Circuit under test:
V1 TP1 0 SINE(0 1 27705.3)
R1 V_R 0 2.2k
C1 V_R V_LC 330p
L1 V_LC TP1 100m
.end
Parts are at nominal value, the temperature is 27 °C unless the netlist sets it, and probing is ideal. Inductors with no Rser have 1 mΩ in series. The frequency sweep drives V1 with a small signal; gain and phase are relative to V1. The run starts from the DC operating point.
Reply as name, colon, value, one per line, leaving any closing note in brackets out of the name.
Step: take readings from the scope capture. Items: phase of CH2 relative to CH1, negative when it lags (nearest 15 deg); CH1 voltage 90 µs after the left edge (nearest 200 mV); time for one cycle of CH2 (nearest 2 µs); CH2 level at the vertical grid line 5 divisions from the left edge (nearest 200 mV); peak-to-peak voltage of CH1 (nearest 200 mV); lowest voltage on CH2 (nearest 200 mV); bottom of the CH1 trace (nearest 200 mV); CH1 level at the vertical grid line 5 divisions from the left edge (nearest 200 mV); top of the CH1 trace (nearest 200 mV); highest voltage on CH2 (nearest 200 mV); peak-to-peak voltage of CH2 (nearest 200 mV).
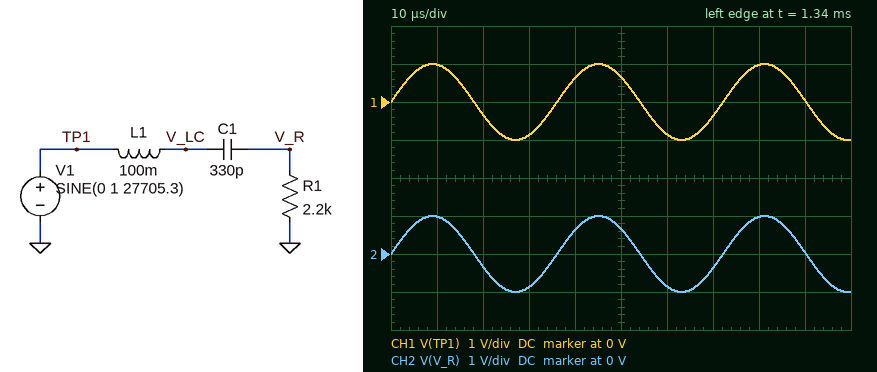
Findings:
phase of CH2 relative to CH1, negative when it lags: 0 deg
CH1 voltage 90 µs after the left edge: 0 V
time for one cycle of CH2: 36 µs
CH2 level at the vertical grid line 5 divisions from the left edge: 600 mV
peak-to-peak voltage of CH1: 2.0 V
lowest voltage on CH2: -1.0 V
bottom of the CH1 trace: -1.0 V
CH1 level at the vertical grid line 5 divisions from the left edge: 600 mV
top of the CH1 trace: 1.0 V
highest voltage on CH2: 1.0 V
peak-to-peak voltage of CH2: 2.0 V
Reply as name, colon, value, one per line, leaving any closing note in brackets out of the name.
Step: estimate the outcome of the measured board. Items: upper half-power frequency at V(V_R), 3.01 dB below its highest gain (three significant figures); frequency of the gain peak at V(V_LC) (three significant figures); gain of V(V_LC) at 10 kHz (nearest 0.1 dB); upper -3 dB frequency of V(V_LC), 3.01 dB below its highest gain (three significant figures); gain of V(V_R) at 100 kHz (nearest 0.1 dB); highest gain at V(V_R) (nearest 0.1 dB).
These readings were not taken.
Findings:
upper half-power frequency at V(V_R), 3.01 dB below its highest gain: 29.5 kHz
frequency of the gain peak at V(V_LC): 27.6 kHz
gain of V(V_LC) at 10 kHz: 1.2 dB
upper -3 dB frequency of V(V_LC), 3.01 dB below its highest gain: 29.3 kHz
gain of V(V_R) at 100 kHz: -28.4 dB
highest gain at V(V_R): 0 dB
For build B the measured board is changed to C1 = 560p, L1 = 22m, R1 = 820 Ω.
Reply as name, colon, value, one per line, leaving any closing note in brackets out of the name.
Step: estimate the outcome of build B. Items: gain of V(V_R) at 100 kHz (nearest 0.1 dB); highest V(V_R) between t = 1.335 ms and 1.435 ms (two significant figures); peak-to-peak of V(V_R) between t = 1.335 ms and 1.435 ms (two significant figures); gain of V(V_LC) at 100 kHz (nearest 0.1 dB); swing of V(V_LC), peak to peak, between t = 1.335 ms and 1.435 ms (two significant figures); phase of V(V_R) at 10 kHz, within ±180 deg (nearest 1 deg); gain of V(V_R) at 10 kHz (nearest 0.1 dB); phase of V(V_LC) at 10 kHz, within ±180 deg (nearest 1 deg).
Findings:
gain of V(V_R) at 100 kHz: -22.6 dB
highest V(V_R) between t = 1.335 ms and 1.435 ms: 130 mV
peak-to-peak of V(V_R) between t = 1.335 ms and 1.435 ms: 250 mV
gain of V(V_LC) at 100 kHz: -11.4 dB
swing of V(V_LC), peak to peak, between t = 1.335 ms and 1.435 ms: 3.2 V
phase of V(V_R) at 10 kHz, within ±180 deg: 88 deg
gain of V(V_R) at 10 kHz: -30.4 dB
phase of V(V_LC) at 10 kHz, within ±180 deg: 0 deg
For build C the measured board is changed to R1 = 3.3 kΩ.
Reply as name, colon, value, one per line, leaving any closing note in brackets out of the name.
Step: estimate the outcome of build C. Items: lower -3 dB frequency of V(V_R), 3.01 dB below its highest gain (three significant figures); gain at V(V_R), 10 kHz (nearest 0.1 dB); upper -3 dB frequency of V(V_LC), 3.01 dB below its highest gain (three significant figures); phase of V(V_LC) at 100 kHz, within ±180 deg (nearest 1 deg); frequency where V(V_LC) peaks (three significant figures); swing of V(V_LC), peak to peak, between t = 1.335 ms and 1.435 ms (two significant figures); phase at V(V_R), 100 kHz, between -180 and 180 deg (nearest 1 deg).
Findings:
lower -3 dB frequency of V(V_R), 3.01 dB below its highest gain: 25.2 kHz
gain at V(V_R), 10 kHz: -22.1 dB
upper -3 dB frequency of V(V_LC), 3.01 dB below its highest gain: 30.0 kHz
phase of V(V_LC) at 100 kHz, within ±180 deg: -142 deg
frequency where V(V_LC) peaks: 27.5 kHz
swing of V(V_LC), peak to peak, between t = 1.335 ms and 1.435 ms: 11 V
phase at V(V_R), 100 kHz, between -180 and 180 deg: -87 deg
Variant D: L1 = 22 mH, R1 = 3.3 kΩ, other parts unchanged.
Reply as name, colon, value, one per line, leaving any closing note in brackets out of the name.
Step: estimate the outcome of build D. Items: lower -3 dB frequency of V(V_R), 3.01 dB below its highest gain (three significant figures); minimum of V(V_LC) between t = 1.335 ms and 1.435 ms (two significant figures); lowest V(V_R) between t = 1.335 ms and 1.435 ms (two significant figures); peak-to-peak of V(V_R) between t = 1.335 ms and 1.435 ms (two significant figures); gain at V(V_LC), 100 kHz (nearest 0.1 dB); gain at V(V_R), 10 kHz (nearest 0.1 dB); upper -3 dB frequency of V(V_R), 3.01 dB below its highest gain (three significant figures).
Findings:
lower -3 dB frequency of V(V_R), 3.01 dB below its highest gain: 48.3 kHz
minimum of V(V_LC) between t = 1.335 ms and 1.435 ms: -1.3 V
lowest V(V_R) between t = 1.335 ms and 1.435 ms: -240 mV
peak-to-peak of V(V_R) between t = 1.335 ms and 1.435 ms: 470 mV
gain at V(V_LC), 100 kHz: -4.3 dB
gain at V(V_R), 10 kHz: -23.1 dB
upper -3 dB frequency of V(V_R), 3.01 dB below its highest gain: 72.2 kHz
